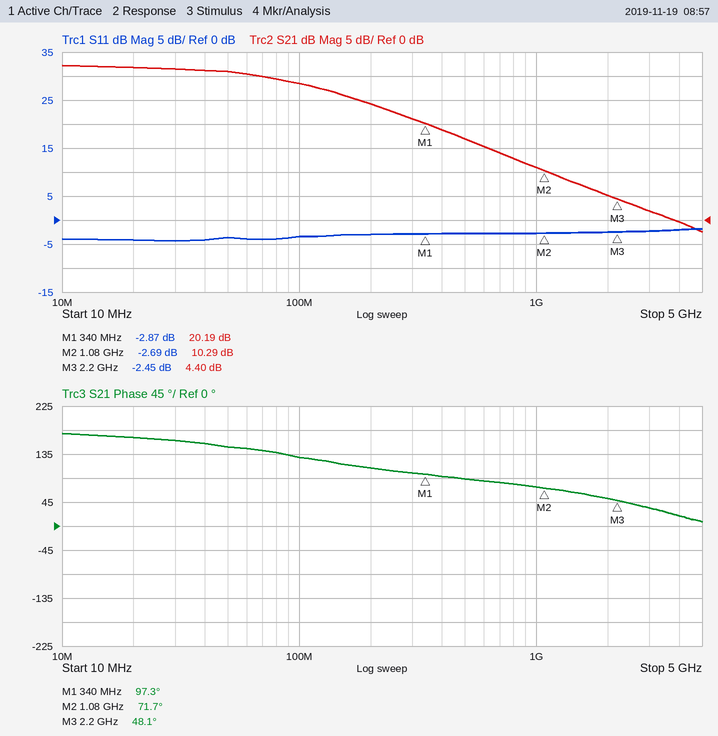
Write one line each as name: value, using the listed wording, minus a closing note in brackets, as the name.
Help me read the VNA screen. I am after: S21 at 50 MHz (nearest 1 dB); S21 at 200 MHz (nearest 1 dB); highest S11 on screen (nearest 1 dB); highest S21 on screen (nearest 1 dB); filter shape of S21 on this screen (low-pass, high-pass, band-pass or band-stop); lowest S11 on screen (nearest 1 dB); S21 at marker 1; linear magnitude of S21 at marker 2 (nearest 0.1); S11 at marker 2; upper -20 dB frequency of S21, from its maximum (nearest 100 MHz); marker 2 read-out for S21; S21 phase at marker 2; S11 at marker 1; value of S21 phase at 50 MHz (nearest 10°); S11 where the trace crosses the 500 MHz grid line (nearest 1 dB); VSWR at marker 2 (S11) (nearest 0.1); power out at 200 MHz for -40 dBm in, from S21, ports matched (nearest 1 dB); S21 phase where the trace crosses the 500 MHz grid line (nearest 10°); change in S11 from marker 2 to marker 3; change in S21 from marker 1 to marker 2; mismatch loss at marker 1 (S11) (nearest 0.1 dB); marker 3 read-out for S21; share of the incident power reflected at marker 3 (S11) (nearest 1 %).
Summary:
S21 at 50 MHz: 31 dB
S21 at 200 MHz: 24 dB
highest S11 on screen: -2 dB
highest S21 on screen: 32 dB
filter shape of S21 on this screen: low-pass
lowest S11 on screen: -4 dB
S21 at marker 1: 20.19 dB
linear magnitude of S21 at marker 2: 3.3
S11 at marker 2: -2.69 dB
upper -20 dB frequency of S21, from its maximum: 900 MHz
marker 2 read-out for S21: 10.29 dB
S21 phase at marker 2: 71.7°
S11 at marker 1: -2.87 dB
value of S21 phase at 50 MHz: 150°
S11 where the trace crosses the 500 MHz grid line: -3 dB
VSWR at marker 2 (S11): 6.5
power out at 200 MHz for -40 dBm in, from S21, ports matched: -16 dBm
S21 phase where the trace crosses the 500 MHz grid line: 90°
change in S11 from marker 2 to marker 3: 0.24 dB
change in S21 from marker 1 to marker 2: -9.90 dB
mismatch loss at marker 1 (S11): 3.2 dB
marker 3 read-out for S21: 4.40 dB
share of the incident power reflected at marker 3 (S11): 57 %
